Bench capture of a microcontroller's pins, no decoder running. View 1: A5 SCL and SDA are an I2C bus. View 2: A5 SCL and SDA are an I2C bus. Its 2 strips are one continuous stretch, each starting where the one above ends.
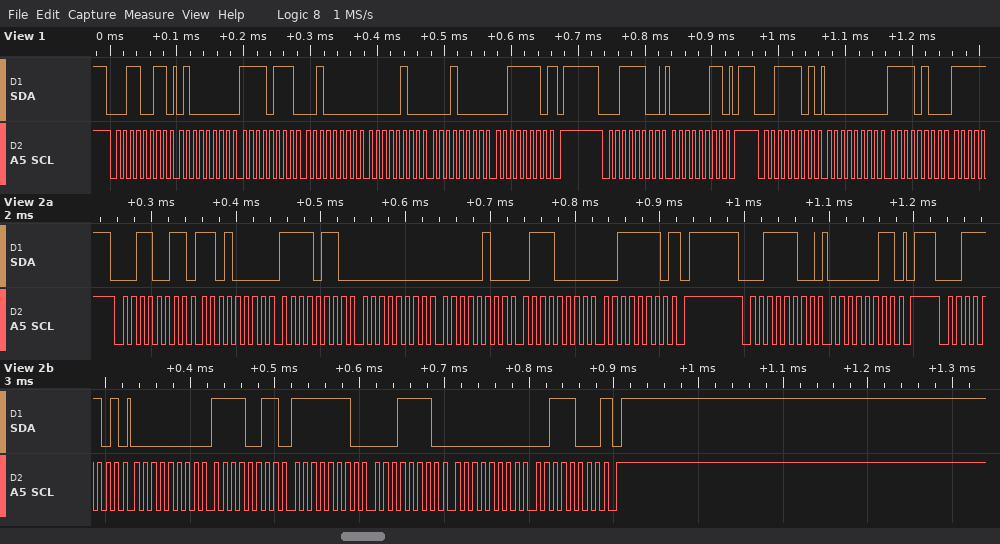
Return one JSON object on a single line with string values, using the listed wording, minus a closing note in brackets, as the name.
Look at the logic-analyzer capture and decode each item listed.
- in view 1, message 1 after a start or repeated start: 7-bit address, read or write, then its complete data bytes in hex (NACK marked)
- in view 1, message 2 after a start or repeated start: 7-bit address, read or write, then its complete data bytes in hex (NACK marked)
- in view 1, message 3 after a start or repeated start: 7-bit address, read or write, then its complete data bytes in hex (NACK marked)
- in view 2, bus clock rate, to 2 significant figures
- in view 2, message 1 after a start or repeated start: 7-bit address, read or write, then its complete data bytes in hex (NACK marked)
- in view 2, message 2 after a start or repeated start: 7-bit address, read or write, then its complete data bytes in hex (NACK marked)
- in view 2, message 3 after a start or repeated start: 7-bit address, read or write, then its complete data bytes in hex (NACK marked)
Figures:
{"in view 1, message 1 after a start or repeated start: 7-bit address, read or write, then its complete data bytes in hex": "0x19 read: 40 F7 20 04 10 3E NACK", "in view 1, message 2 after a start or repeated start: 7-bit address, read or write, then its complete data bytes in hex": "0x1E write: 03", "in view 1, message 3 after a start or repeated start: 7-bit address, read or write, then its complete data bytes in hex": "0x1E read: 00 F4", "in view 2, bus clock rate, to 2 significant figures": "100 kHz", "in view 2, message 1 after a start or repeated start: 7-bit address, read or write, then its complete data bytes in hex": "0x19 read: D0 F6 00 04 70 3E NACK", "in view 2, message 2 after a start or repeated start: 7-bit address, read or write, then its complete data bytes in hex": "0x1E write: 03", "in view 2, message 3 after a start or repeated start: 7-bit address, read or write, then its complete data bytes in hex": "0x1E read: 00 F3 FE 1E 00 38 NACK"}
